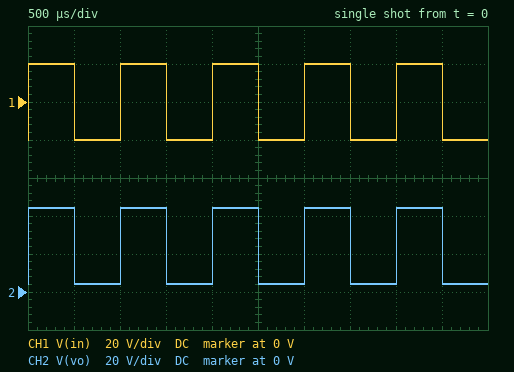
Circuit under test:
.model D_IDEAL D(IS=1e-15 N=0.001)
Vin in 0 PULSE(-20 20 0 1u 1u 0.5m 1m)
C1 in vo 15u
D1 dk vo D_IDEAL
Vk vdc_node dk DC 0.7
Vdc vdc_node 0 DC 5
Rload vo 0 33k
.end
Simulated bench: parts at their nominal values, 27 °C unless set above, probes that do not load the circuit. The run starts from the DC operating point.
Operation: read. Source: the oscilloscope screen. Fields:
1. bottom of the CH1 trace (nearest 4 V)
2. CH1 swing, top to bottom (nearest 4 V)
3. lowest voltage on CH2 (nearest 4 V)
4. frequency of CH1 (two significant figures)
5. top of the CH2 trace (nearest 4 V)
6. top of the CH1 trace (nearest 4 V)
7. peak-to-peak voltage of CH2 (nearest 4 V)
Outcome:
-20 V
40 V
4 V
1.0 kHz
44 V
20 V
40 V
